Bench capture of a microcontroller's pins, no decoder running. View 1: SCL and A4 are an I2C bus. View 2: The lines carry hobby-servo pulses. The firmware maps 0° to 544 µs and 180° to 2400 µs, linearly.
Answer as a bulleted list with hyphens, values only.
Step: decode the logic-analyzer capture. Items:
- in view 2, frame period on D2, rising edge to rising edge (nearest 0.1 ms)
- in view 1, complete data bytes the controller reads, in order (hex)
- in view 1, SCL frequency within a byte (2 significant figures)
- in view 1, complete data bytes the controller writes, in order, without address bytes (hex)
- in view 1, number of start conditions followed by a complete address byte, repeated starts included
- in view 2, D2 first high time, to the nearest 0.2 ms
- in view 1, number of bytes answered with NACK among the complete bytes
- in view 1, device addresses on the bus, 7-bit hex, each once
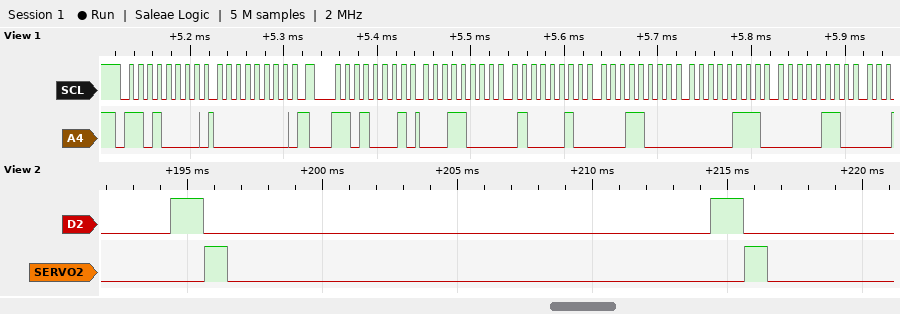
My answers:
- 20.0 ms
- 18 42 18 07 06
- 100 kHz
- 00
- 2
- 1.2 ms
- 0
- 0x68
